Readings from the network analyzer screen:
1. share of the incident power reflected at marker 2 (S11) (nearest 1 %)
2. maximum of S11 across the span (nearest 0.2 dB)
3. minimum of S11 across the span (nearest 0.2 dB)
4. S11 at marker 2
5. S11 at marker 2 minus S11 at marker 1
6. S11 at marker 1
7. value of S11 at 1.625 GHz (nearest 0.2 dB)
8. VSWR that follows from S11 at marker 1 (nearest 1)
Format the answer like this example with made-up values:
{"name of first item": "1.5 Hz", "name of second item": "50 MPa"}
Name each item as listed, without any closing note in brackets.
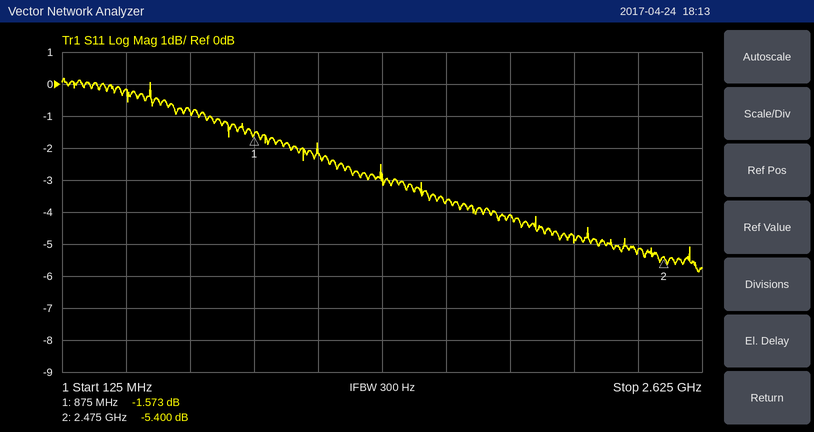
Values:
{"share of the incident power reflected at marker 2 (S11)": "29 %", "maximum of S11 across the span": "0.2 dB", "minimum of S11 across the span": "-5.8 dB", "S11 at marker 2": "-5.400 dB", "S11 at marker 2 minus S11 at marker 1": "-3.827 dB", "S11 at marker 1": "-1.573 dB", "value of S11 at 1.625 GHz": "-3.6 dB", "VSWR that follows from S11 at marker 1": "11"}
